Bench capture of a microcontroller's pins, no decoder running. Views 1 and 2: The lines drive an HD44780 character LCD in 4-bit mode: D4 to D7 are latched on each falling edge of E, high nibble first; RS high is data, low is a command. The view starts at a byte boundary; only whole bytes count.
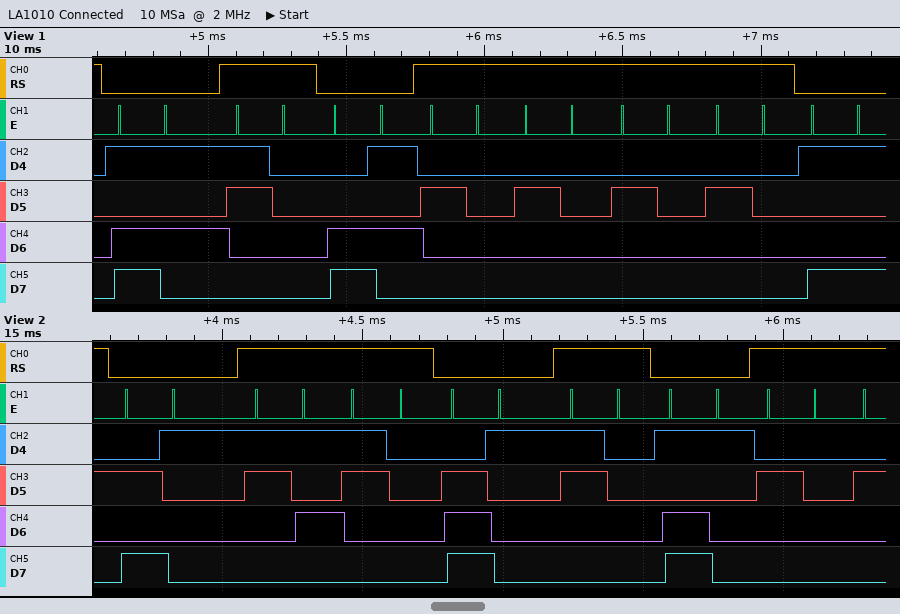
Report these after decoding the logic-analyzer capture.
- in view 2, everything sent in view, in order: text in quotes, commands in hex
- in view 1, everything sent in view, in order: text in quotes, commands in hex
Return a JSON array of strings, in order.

["0xA1 \"50\" 0xE1 \"0\" 0xD1 \" \"", "0xD5 \"0\" 0xC5 \"    \" 0x99"]
